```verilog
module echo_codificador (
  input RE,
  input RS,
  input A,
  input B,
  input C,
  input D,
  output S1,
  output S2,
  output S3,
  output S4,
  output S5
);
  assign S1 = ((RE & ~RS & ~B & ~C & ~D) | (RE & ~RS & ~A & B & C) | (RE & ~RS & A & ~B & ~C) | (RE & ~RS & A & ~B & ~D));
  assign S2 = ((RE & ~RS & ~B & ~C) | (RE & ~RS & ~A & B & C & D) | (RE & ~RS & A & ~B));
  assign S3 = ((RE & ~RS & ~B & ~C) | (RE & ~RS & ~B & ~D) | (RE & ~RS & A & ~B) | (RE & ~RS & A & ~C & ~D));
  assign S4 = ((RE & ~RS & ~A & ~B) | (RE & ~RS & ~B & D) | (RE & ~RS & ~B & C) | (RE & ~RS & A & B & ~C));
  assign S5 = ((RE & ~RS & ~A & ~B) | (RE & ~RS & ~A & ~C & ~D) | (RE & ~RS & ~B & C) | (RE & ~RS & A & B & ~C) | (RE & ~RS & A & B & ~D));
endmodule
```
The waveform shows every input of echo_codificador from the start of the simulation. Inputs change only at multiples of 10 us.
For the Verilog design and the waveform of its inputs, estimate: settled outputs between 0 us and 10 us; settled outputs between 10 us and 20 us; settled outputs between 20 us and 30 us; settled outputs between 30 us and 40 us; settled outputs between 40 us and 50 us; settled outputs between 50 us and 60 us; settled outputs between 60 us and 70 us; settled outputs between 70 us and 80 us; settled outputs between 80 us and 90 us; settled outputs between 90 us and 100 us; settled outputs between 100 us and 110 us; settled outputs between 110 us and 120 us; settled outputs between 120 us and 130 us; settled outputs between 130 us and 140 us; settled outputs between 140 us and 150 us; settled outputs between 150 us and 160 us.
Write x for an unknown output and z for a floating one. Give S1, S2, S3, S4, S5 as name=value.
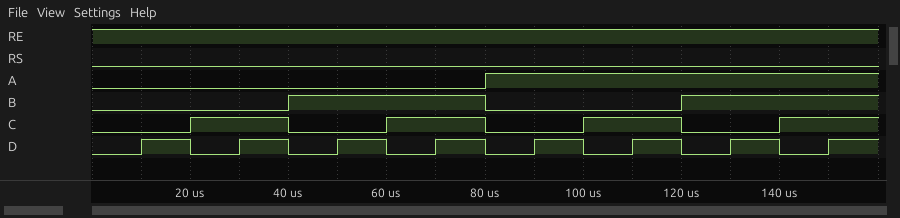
S1=1, S2=1, S3=1, S4=1, S5=1
S1=0, S2=1, S3=1, S4=1, S5=1
S1=0, S2=0, S3=1, S4=1, S5=1
S1=0, S2=0, S3=0, S4=1, S5=1
S1=0, S2=0, S3=0, S4=0, S5=1
S1=0, S2=0, S3=0, S4=0, S5=0
S1=1, S2=0, S3=0, S4=0, S5=0
S1=1, S2=1, S3=0, S4=0, S5=0
S1=1, S2=1, S3=1, S4=0, S5=0
S1=1, S2=1, S3=1, S4=1, S5=0
S1=1, S2=1, S3=1, S4=1, S5=1
S1=0, S2=1, S3=1, S4=1, S5=1
S1=0, S2=0, S3=1, S4=1, S5=1
S1=0, S2=0, S3=0, S4=1, S5=1
S1=0, S2=0, S3=0, S4=0, S5=1
S1=0, S2=0, S3=0, S4=0, S5=0
